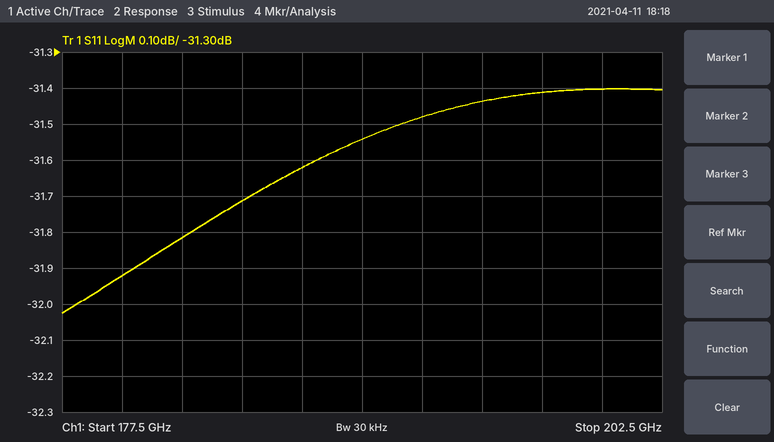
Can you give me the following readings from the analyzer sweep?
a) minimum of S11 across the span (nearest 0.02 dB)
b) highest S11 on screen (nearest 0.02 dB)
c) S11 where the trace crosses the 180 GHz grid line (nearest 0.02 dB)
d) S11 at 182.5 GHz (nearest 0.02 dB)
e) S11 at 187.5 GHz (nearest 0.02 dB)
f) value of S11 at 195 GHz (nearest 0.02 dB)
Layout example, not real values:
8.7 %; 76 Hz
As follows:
-32.02 dB; -31.40 dB; -31.92 dB; -31.82 dB; -31.62 dB; -31.44 dB
